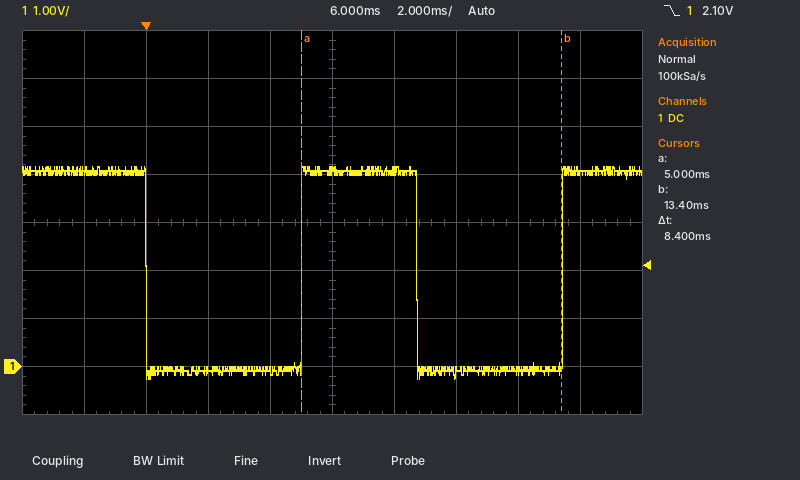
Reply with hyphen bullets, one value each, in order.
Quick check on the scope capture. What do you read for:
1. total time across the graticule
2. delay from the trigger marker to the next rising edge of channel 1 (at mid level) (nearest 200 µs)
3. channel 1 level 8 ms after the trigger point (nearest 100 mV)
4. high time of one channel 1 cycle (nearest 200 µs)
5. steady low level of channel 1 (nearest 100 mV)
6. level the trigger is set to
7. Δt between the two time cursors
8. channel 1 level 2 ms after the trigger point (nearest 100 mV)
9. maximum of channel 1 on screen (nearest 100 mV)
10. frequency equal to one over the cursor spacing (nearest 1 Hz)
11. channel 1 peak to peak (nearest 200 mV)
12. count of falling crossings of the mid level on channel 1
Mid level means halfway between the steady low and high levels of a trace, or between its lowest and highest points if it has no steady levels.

- 20 ms
- 5.0 ms
- 4.1 V
- 3.8 ms
- -100 mV
- 2.10 V
- 8.4 ms
- -100 mV
- 4.2 V
- 119 Hz
- 4.4 V
- 2
